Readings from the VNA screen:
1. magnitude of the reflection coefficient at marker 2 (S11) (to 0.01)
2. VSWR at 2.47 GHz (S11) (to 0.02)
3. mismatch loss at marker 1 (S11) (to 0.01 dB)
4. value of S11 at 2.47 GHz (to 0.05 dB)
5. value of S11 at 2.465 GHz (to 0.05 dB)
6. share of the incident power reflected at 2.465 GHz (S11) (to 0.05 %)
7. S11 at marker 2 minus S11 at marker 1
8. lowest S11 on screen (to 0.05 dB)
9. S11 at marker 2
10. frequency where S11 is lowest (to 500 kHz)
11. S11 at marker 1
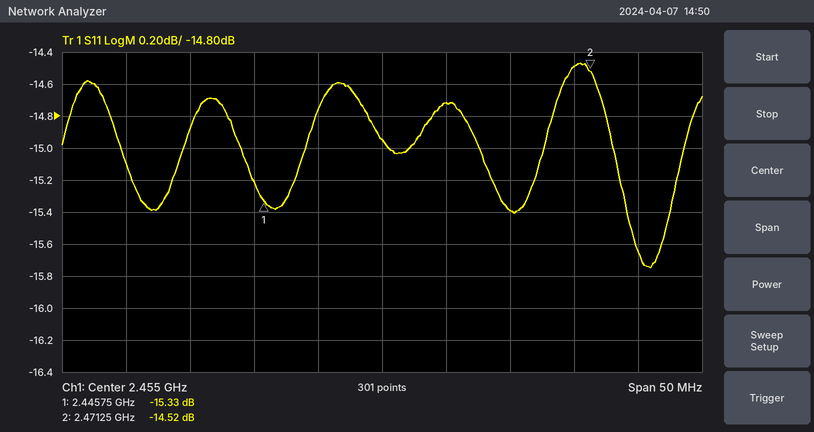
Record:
0.19
1.46
0.13 dB
-14.50 dB
-15.40 dB
2.90 %
0.81 dB
-15.75 dB
-14.52 dB
2.4760 GHz
-15.33 dB
